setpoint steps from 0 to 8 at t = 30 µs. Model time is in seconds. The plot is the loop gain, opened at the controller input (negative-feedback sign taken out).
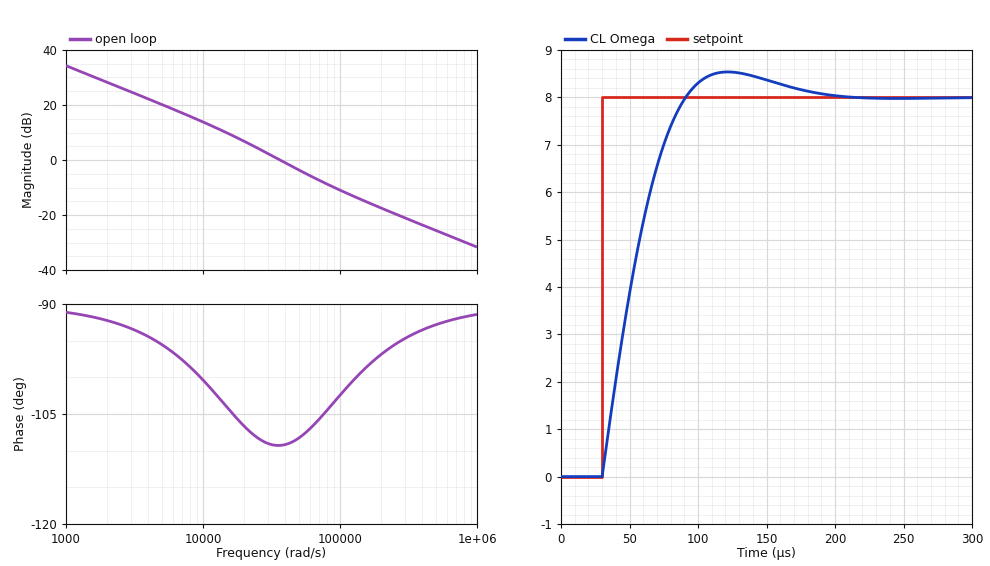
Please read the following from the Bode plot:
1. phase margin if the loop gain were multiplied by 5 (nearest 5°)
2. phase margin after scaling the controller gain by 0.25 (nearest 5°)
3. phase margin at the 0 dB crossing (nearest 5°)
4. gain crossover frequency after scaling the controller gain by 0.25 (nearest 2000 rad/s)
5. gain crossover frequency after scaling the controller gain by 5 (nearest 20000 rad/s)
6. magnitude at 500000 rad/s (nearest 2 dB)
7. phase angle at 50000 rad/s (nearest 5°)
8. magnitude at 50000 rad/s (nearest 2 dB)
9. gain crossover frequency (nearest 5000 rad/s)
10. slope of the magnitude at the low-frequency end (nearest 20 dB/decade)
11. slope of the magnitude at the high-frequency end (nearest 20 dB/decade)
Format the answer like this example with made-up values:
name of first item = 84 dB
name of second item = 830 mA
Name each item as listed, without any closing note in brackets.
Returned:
phase margin if the loop gain were multiplied by 5 = 80°
phase margin after scaling the controller gain by 0.25 = 80°
phase margin at the 0 dB crossing = 70°
gain crossover frequency after scaling the controller gain by 0.25 = 12000 rad/s
gain crossover frequency after scaling the controller gain by 5 = 140000 rad/s
magnitude at 500000 rad/s = -26 dB
phase angle at 50000 rad/s = -110°
magnitude at 50000 rad/s = -4 dB
gain crossover frequency = 35000 rad/s
slope of the magnitude at the low-frequency end = -20 dB/decade
slope of the magnitude at the high-frequency end = -20 dB/decade
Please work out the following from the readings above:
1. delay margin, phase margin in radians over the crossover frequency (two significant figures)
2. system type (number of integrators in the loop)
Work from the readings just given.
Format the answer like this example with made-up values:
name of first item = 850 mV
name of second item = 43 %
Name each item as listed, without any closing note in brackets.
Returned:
delay margin, phase margin in radians over the crossover frequency = 0.000035 s
system type = 1
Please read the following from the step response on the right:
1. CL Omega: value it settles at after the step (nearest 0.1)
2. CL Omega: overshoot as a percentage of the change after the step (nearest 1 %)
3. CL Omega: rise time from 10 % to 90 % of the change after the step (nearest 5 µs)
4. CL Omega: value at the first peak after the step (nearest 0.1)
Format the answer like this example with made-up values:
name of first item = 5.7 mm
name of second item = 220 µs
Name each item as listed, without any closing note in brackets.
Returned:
CL Omega: value it settles at after the step = 8.0
CL Omega: overshoot as a percentage of the change after the step = 7 %
CL Omega: rise time from 10 % to 90 % of the change after the step = 45 µs
CL Omega: value at the first peak after the step = 8.5
